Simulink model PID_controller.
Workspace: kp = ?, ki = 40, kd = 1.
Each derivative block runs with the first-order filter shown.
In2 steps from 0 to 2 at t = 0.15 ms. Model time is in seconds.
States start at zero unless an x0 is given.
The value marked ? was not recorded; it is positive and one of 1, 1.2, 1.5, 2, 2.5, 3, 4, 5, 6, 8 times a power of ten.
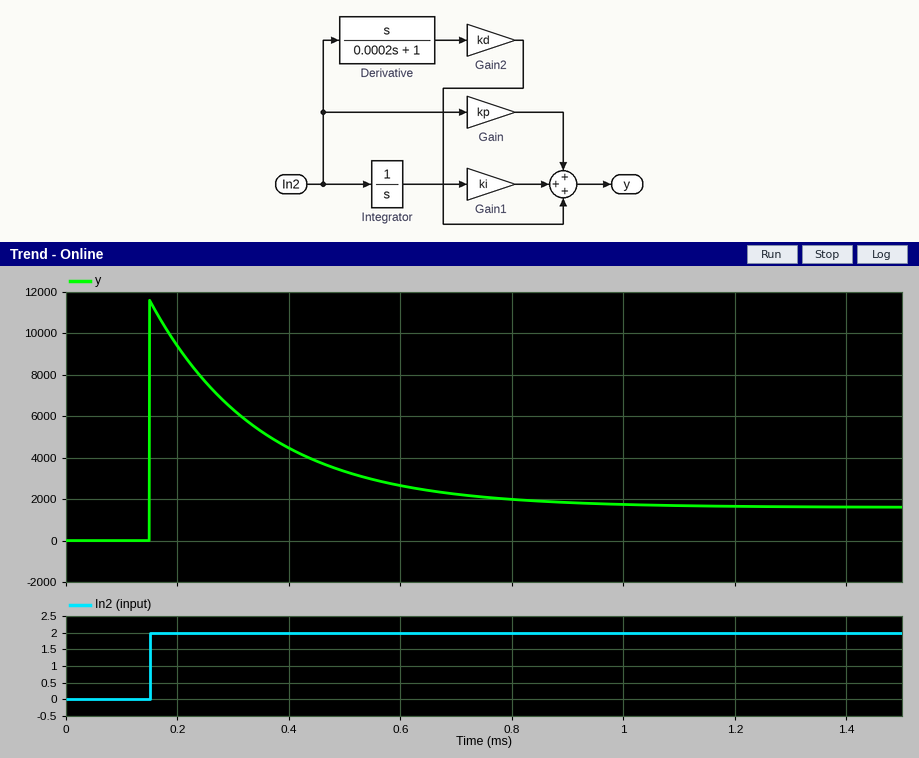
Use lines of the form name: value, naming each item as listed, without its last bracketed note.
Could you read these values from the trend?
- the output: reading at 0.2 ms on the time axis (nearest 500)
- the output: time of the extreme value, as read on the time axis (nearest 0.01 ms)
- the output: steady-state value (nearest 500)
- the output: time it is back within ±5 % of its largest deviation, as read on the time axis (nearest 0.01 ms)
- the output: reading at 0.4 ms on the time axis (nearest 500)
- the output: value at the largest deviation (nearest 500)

the output: reading at 0.2 ms on the time axis: 9500
the output: time of the extreme value, as read on the time axis: 0.15 ms
the output: steady-state value: 1500
the output: time it is back within ±5 % of its largest deviation, as read on the time axis: 0.72 ms
the output: reading at 0.4 ms on the time axis: 4500
the output: value at the largest deviation: 11500
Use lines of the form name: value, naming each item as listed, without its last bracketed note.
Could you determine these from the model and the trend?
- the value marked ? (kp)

the value marked ?: 800
